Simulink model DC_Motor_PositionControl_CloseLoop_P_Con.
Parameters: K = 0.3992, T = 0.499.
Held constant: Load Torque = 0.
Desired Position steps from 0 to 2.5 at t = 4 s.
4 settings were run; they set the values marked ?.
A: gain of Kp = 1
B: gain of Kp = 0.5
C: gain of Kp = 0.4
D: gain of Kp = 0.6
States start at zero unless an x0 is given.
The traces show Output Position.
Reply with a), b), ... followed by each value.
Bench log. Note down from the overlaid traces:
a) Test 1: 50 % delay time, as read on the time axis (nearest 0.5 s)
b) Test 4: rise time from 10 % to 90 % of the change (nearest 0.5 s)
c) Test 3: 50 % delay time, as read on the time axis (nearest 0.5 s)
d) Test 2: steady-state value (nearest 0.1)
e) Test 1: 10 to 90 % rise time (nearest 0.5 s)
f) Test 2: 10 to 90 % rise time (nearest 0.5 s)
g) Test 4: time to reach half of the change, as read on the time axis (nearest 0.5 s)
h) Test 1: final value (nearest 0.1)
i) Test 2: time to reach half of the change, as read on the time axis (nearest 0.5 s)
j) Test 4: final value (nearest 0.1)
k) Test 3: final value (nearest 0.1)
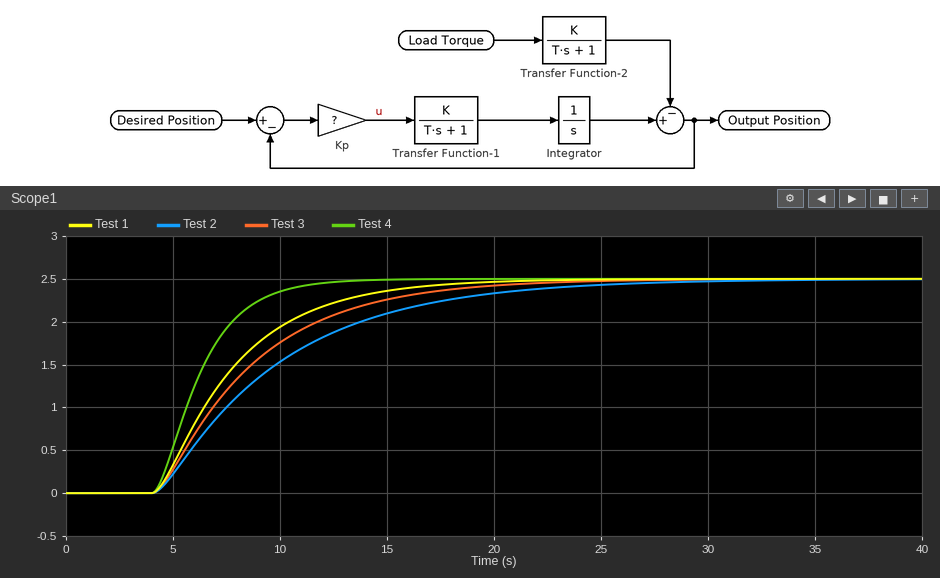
a) 7.0 s
b) 4.5 s
c) 7.5 s
d) 2.5
e) 8.0 s
f) 12.5 s
g) 6.0 s
h) 2.5
i) 8.5 s
j) 2.5
k) 2.5
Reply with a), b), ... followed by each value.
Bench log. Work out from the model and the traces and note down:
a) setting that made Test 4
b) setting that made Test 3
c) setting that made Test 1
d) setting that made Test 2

a) A
b) B
c) D
d) C
